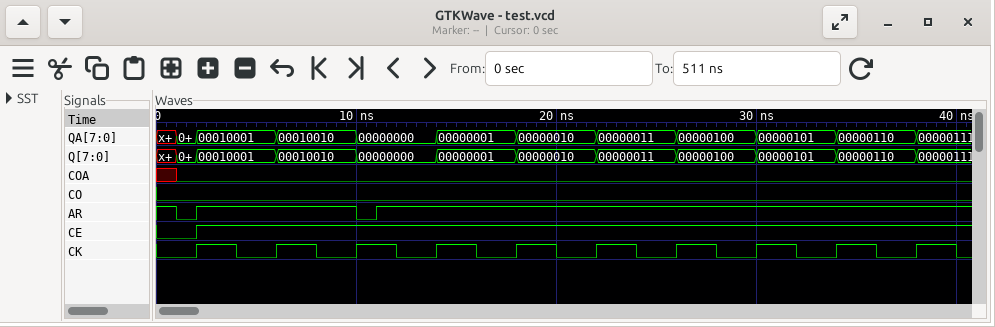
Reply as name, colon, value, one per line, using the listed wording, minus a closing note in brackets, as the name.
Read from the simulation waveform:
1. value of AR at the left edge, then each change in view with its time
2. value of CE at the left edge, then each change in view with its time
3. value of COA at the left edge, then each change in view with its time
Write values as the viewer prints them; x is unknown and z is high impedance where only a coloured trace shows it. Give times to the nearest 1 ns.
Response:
value of AR at the left edge, then each change in view with its time: 1, 0 at 1 ns, 1 at 2 ns, 0 at 10 ns, 1 at 11 ns
value of CE at the left edge, then each change in view with its time: 0, 1 at 2 ns
value of COA at the left edge, then each change in view with its time: x, 0 at 1 ns
